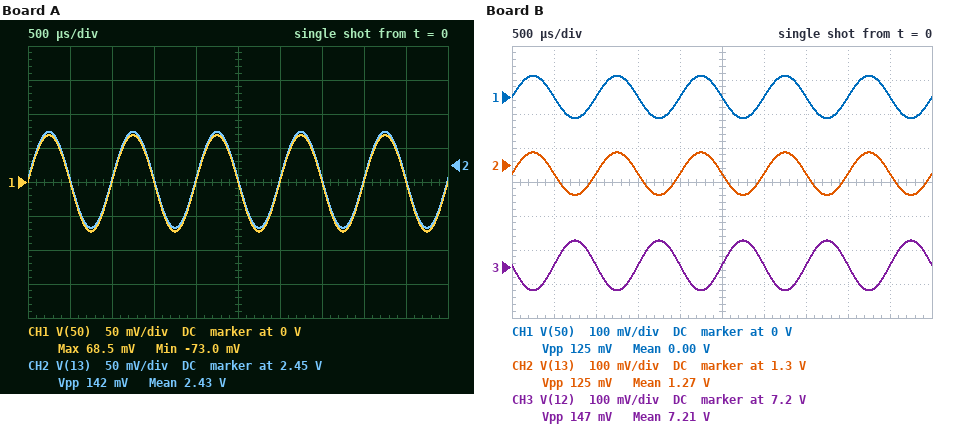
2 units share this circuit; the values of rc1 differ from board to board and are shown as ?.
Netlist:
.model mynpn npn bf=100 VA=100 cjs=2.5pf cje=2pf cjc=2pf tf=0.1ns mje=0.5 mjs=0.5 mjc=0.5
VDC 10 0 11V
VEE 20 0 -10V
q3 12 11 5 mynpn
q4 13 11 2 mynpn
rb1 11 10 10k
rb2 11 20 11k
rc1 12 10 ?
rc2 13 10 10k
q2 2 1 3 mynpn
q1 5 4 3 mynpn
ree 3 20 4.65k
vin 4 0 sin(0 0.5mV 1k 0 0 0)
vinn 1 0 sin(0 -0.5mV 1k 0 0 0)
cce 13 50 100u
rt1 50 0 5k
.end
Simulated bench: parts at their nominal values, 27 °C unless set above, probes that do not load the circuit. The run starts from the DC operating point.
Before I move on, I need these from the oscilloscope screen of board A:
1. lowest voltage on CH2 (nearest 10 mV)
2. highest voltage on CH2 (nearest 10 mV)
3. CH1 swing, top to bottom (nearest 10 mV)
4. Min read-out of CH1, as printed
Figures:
2.36 V
2.50 V
140 mV
-73.0 mV
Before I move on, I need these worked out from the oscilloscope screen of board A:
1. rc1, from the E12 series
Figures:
18 kΩ
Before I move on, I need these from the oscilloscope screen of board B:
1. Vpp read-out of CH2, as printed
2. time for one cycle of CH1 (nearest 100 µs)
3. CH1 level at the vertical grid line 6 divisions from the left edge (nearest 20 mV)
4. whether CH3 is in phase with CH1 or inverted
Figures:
125 mV
1.0 ms
0 V
inverted
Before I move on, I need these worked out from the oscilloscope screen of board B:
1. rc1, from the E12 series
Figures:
3.9 kΩ
